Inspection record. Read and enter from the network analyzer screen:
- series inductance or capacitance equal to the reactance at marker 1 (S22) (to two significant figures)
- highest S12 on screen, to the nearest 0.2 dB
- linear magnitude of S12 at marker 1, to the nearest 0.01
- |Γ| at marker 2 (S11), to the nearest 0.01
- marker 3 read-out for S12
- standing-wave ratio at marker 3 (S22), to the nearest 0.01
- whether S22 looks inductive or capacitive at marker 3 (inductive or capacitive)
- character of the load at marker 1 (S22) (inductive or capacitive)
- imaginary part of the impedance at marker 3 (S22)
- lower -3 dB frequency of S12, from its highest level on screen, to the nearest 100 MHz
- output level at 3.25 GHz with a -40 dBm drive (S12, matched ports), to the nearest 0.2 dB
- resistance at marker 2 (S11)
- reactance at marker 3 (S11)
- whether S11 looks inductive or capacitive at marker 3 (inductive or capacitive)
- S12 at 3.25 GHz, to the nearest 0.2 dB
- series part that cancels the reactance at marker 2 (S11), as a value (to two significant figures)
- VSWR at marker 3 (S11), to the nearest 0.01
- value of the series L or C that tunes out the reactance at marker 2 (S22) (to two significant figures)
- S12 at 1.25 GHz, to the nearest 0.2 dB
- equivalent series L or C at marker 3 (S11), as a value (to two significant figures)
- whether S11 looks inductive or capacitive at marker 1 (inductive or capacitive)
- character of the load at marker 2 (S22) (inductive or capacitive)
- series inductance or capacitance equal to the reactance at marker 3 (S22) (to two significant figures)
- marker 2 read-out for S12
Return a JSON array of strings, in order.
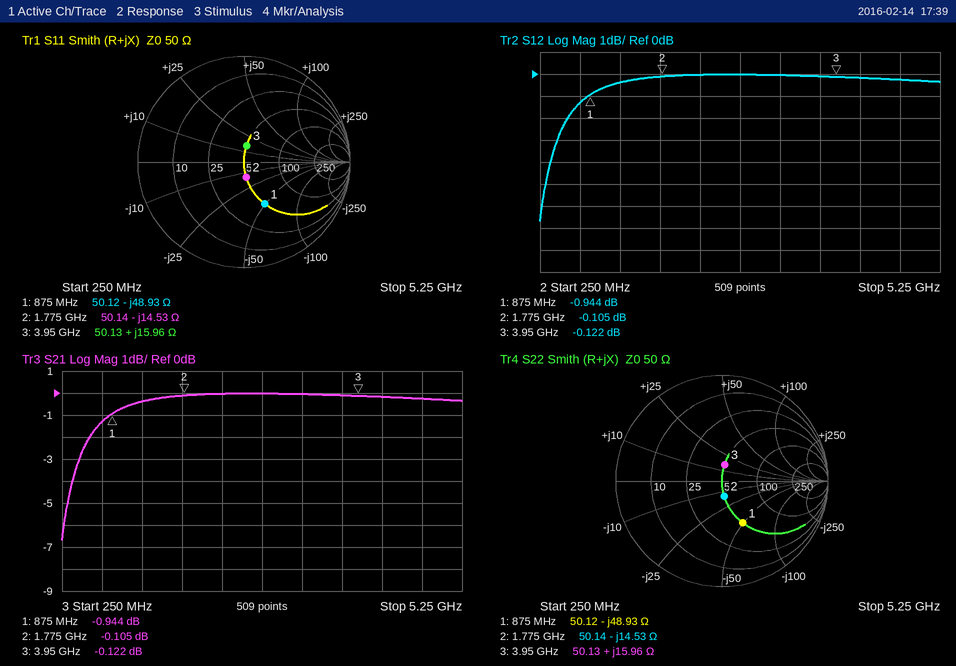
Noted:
["3.7 pF", "0.0 dB", "0.90", "0.14", "-0.122 dB", "1.37", "inductive", "capacitive", "+15.96 Ω", "500 MHz", "-40.0 dBm", "50.14 Ω", "+15.96 Ω", "inductive", "0.0 dB", "1.3 nH", "1.37", "1.3 nH", "-0.4 dB", "640 pH", "capacitive", "capacitive", "640 pH", "-0.105 dB"]
